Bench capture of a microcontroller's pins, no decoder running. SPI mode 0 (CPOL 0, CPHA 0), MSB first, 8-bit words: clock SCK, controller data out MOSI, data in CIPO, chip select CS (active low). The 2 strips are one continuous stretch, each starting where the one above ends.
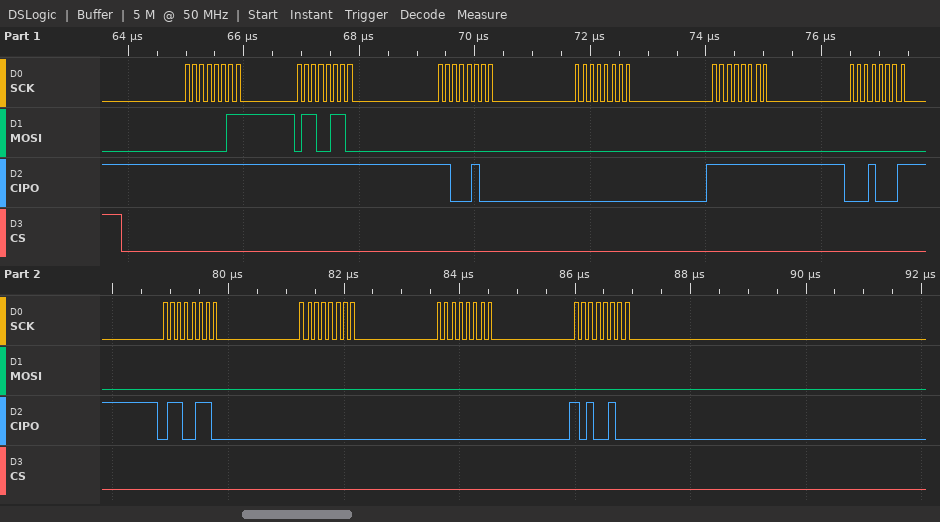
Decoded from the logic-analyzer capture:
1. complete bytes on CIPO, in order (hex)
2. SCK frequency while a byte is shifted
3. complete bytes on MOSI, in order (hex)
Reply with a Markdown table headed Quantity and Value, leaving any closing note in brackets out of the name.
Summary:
| Quantity | Value |
|---|---|
| complete bytes on CIPO, in order | FF FF C4 00 FF 11 66 00 00 A4 |
| SCK frequency while a byte is shifted | 8 MHz |
| complete bytes on MOSI, in order | 03 66 00 00 00 00 00 00 00 00 |
